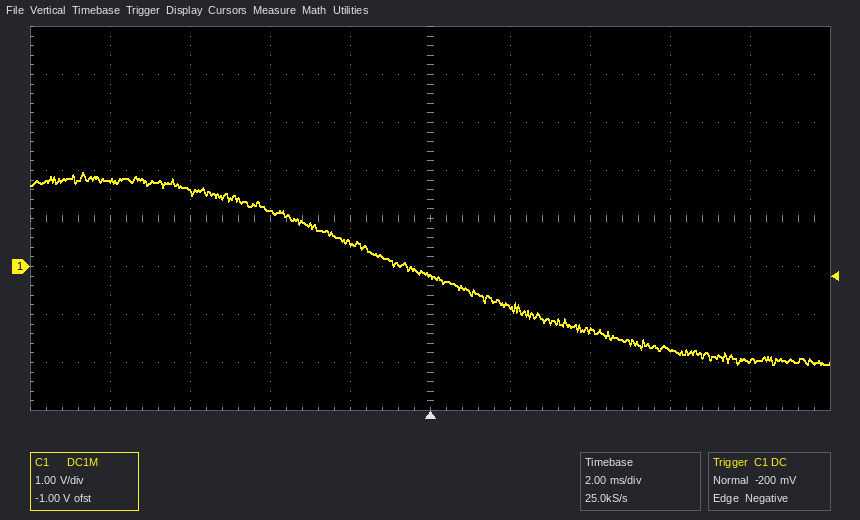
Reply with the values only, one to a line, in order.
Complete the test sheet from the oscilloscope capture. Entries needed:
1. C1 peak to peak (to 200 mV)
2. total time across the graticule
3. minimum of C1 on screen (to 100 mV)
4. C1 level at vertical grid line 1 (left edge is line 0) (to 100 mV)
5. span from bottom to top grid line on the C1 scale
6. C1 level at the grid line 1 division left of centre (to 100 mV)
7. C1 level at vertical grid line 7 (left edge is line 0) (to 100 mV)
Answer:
4.0 V
20 ms
-2.0 V
1.8 V
8 V
500 mV
-1.3 V
